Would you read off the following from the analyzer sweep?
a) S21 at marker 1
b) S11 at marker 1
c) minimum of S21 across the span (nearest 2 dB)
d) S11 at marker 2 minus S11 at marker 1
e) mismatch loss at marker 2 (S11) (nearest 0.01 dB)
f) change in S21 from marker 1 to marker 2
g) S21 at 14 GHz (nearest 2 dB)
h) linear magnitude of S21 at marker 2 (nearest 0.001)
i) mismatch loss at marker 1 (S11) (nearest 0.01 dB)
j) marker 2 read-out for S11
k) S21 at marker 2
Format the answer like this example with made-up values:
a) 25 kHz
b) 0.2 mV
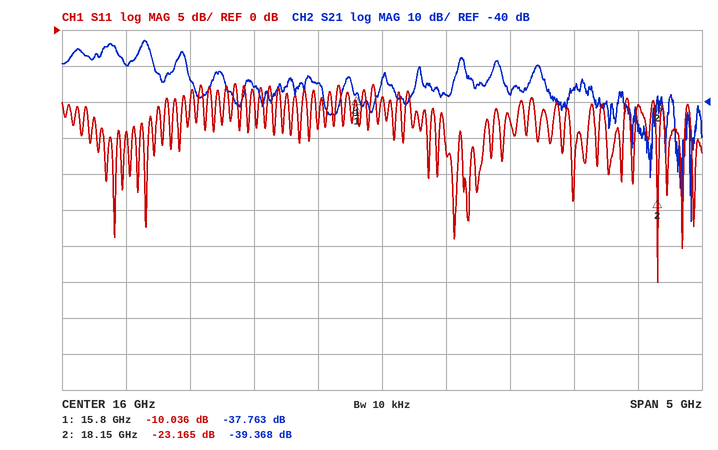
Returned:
a) -37.763 dB
b) -10.036 dB
c) -74 dB
d) -13.129 dB
e) 0.02 dB
f) -1.605 dB
g) -30 dB
h) 0.011
i) 0.45 dB
j) -23.165 dB
k) -39.368 dB
